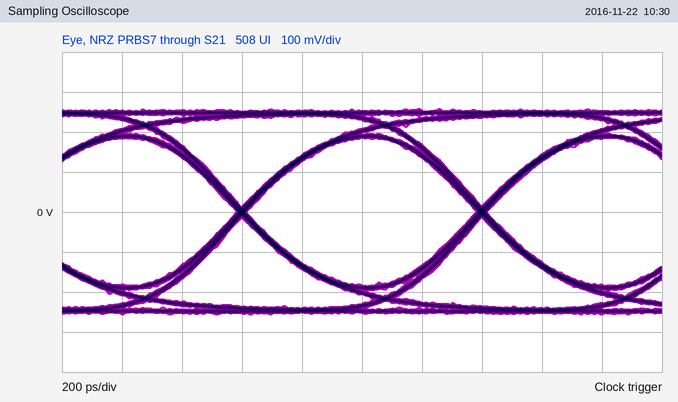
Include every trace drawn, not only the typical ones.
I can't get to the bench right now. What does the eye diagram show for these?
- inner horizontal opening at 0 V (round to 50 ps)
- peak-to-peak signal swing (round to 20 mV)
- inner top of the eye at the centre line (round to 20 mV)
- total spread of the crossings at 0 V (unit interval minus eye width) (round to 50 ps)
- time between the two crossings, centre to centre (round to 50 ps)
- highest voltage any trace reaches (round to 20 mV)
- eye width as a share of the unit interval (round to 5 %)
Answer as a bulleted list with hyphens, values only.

- 750 ps
- 520 mV
- 180 mV
- 50 ps
- 800 ps
- 260 mV
- 95 %
